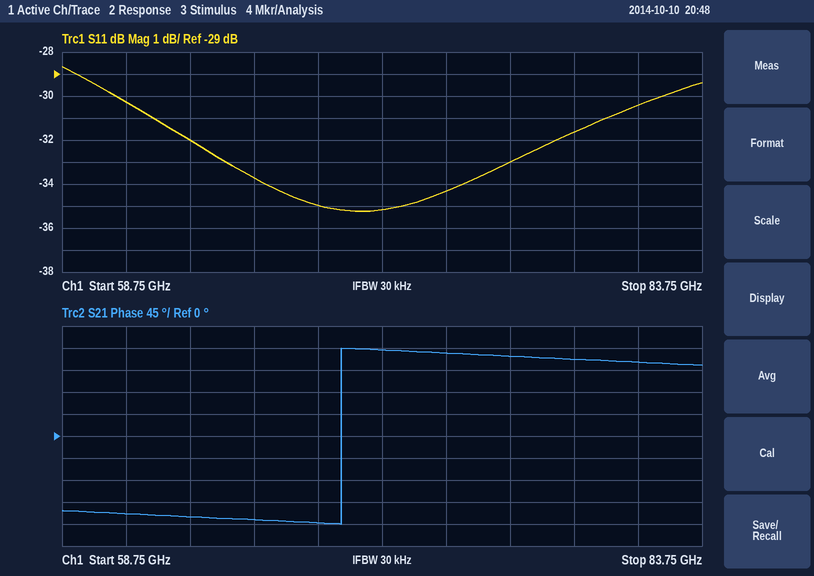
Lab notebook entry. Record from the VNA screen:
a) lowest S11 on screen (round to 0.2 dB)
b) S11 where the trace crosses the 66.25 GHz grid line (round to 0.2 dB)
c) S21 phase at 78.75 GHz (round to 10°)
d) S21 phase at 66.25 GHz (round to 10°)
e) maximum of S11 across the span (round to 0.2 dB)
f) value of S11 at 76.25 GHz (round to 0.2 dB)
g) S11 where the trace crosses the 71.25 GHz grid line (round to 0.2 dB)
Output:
-35.2 dB
-33.8 dB
160°
-170°
-28.6 dB
-33.0 dB
-35.2 dB
